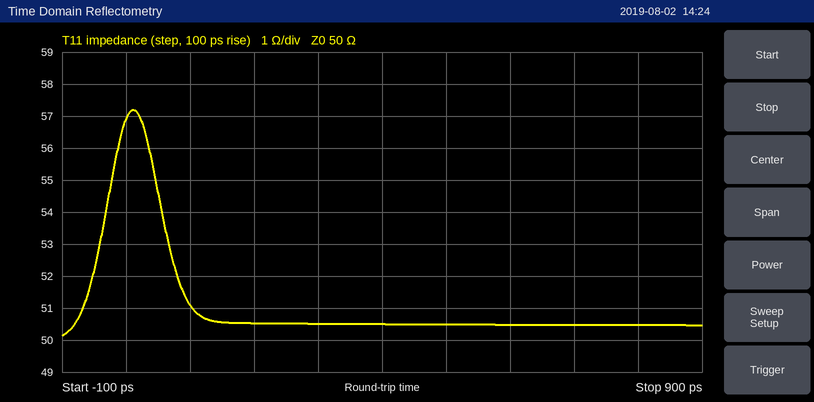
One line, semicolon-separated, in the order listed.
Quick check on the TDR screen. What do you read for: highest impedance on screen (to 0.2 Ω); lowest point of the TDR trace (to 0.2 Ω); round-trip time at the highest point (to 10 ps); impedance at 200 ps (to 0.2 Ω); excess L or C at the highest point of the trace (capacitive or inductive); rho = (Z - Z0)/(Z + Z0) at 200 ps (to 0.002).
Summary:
57.2 Ω; 50.2 Ω; 10 ps; 50.6 Ω; inductive; +0.006
